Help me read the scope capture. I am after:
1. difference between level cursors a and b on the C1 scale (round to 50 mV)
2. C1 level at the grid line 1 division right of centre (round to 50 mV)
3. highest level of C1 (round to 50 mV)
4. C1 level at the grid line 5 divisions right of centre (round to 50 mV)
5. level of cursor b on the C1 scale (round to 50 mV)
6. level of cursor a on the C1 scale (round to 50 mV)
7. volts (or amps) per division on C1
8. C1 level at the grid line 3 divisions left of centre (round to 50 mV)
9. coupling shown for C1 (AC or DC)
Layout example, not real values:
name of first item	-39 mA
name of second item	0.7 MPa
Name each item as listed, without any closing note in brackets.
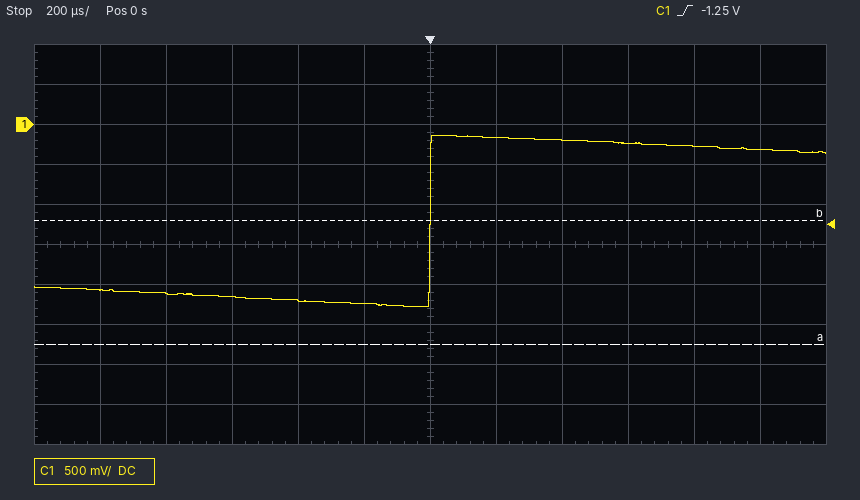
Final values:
difference between level cursors a and b on the C1 scale	1.55 V
C1 level at the grid line 1 division right of centre	-150 mV
highest level of C1	-150 mV
C1 level at the grid line 5 divisions right of centre	-300 mV
level of cursor b on the C1 scale	-1.20 V
level of cursor a on the C1 scale	-2.75 V
volts (or amps) per division on C1	500 mV
C1 level at the grid line 3 divisions left of centre	-2.15 V
coupling shown for C1	DC
